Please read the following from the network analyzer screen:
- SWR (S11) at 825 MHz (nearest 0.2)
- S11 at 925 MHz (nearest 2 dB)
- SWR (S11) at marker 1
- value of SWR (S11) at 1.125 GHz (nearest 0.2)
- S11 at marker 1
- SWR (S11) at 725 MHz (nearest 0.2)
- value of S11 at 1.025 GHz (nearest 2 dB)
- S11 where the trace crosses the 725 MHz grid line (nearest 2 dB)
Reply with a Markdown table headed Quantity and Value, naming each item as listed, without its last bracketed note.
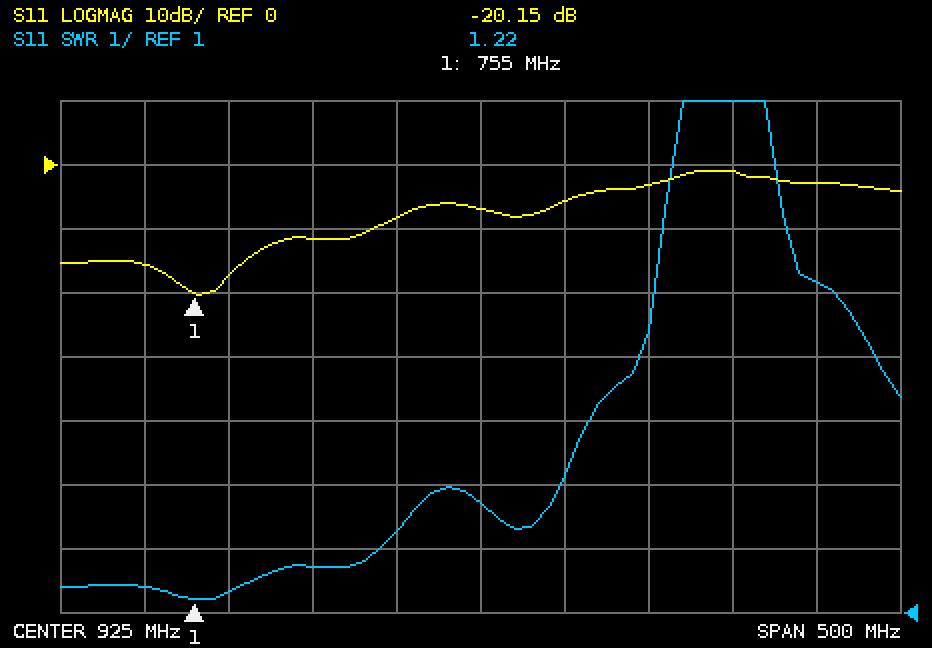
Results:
| Quantity | Value |
|---|---|
| SWR (S11) at 825 MHz | 1.8 |
| S11 at 925 MHz | -6 dB |
| SWR (S11) at marker 1 | 1.22 |
| value of SWR (S11) at 1.125 GHz | 6.2 |
| S11 at marker 1 | -20.15 dB |
| SWR (S11) at 725 MHz | 1.4 |
| value of S11 at 1.025 GHz | -4 dB |
| S11 where the trace crosses the 725 MHz grid line | -16 dB |
